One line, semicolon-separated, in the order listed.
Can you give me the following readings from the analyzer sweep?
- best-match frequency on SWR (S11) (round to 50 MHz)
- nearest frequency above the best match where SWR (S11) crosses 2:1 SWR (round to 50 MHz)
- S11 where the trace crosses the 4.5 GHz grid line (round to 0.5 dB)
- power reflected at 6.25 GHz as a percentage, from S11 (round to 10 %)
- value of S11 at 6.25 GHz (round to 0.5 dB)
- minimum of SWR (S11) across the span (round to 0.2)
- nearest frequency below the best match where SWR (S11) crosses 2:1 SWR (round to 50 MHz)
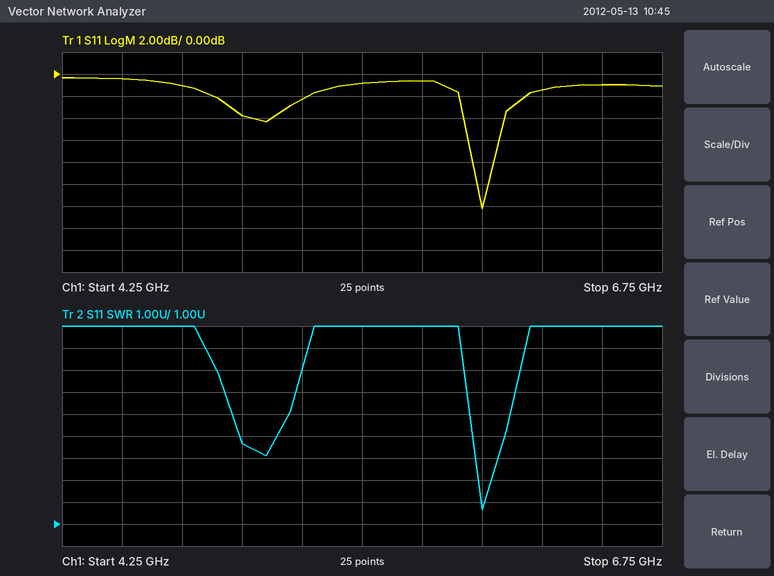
6.00 GHz; 6.00 GHz; -0.5 dB; 70 %; -1.5 dB; 1.6; 6.00 GHz
